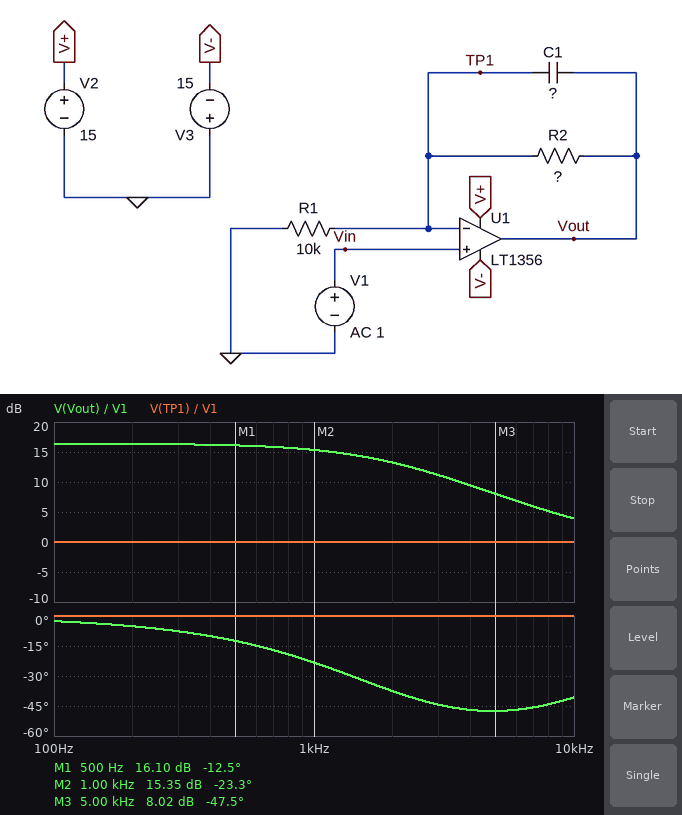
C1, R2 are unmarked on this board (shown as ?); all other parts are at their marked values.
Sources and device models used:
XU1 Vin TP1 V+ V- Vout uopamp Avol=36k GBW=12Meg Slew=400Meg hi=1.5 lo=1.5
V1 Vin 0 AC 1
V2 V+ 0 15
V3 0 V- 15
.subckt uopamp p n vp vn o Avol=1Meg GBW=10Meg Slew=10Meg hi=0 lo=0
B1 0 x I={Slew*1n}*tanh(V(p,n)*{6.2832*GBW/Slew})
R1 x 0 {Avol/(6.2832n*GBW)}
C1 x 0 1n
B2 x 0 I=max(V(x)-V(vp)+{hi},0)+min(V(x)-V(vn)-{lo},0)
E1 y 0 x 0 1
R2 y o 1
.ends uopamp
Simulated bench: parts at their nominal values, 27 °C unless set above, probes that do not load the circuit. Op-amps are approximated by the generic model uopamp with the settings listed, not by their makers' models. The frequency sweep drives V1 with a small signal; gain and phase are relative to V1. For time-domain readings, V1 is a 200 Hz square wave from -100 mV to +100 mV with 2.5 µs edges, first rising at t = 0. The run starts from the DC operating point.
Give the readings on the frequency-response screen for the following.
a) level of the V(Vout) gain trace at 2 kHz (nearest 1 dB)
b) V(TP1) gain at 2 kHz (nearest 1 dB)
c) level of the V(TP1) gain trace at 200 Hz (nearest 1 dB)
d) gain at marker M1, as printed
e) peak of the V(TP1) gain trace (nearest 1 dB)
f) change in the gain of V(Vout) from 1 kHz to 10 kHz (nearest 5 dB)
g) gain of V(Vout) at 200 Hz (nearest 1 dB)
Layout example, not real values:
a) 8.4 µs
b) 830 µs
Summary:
a) 13 dB
b) 0 dB
c) 0 dB
d) 16.10 dB
e) 0 dB
f) -10 dB
g) 16 dB
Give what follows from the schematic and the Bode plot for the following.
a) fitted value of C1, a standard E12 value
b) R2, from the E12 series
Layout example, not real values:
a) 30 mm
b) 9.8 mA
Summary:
a) 1.5 nF
b) 56 kΩ
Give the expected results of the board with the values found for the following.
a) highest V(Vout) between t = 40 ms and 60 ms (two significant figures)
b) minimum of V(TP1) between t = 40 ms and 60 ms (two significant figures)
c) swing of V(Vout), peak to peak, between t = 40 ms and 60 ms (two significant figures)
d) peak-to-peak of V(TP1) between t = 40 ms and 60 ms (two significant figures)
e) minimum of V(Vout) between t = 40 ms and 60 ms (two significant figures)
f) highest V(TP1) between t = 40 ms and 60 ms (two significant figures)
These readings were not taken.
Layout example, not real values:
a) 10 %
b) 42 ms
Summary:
a) 660 mV
b) -100 mV
c) 1.3 V
d) 200 mV
e) -660 mV
f) 100 mV
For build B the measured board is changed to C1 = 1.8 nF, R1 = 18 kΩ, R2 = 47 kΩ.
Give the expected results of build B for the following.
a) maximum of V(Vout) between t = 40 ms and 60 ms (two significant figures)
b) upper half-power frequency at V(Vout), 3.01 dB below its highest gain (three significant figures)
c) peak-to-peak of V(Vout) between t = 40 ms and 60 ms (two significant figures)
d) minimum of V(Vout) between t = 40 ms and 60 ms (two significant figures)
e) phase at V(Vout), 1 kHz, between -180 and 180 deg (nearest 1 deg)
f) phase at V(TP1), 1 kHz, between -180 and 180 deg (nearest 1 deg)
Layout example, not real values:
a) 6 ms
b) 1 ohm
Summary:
a) 360 mV
b) 2.04 kHz
c) 720 mV
d) -360 mV
e) -20 deg
f) 0 deg
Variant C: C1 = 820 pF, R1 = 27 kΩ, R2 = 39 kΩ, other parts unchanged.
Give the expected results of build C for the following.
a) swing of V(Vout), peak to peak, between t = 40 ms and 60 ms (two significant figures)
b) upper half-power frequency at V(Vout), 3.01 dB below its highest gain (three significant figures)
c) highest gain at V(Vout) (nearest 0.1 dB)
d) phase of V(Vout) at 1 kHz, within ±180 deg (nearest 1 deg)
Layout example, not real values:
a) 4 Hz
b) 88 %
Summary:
a) 490 mV
b) 6.10 kHz
c) 7.8 dB
d) -7 deg
